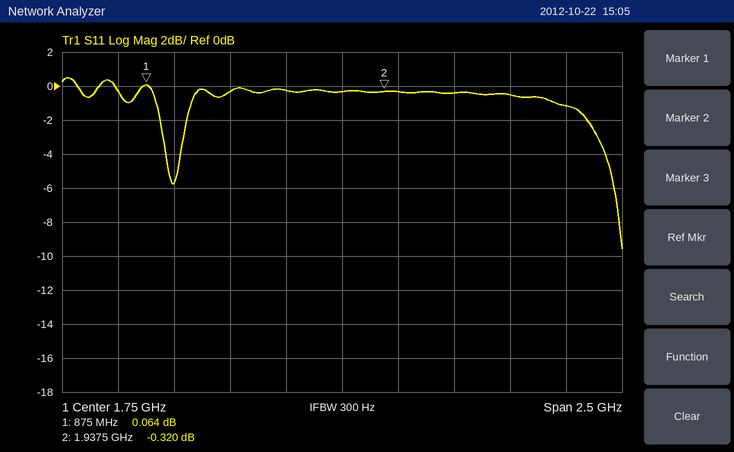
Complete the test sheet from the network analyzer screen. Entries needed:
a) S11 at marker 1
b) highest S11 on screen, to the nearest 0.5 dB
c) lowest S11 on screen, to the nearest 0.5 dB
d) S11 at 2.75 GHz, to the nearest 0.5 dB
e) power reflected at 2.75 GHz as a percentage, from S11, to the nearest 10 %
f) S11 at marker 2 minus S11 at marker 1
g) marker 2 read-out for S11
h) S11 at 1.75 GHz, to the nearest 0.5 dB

0.064 dB
0.5 dB
-9.5 dB
-1.0 dB
80 %
-0.384 dB
-0.320 dB
-0.5 dB
